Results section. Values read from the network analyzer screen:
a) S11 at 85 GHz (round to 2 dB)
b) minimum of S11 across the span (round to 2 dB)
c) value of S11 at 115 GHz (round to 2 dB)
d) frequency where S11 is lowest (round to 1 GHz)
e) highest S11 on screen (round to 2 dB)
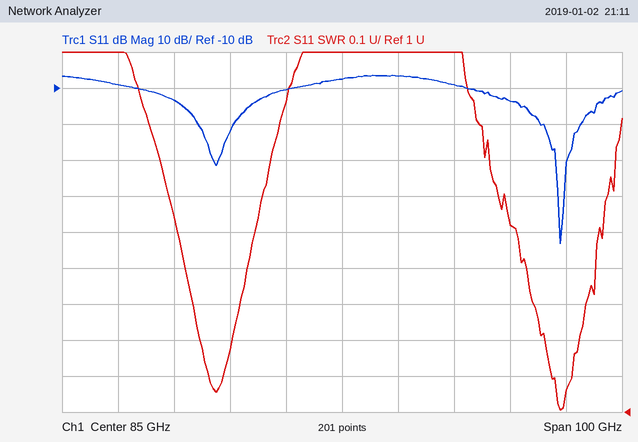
-8 dB
-54 dB
-14 dB
124 GHz
-6 dB
